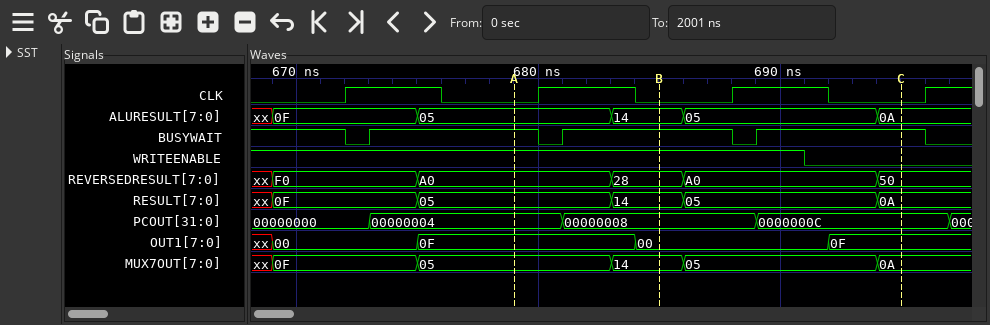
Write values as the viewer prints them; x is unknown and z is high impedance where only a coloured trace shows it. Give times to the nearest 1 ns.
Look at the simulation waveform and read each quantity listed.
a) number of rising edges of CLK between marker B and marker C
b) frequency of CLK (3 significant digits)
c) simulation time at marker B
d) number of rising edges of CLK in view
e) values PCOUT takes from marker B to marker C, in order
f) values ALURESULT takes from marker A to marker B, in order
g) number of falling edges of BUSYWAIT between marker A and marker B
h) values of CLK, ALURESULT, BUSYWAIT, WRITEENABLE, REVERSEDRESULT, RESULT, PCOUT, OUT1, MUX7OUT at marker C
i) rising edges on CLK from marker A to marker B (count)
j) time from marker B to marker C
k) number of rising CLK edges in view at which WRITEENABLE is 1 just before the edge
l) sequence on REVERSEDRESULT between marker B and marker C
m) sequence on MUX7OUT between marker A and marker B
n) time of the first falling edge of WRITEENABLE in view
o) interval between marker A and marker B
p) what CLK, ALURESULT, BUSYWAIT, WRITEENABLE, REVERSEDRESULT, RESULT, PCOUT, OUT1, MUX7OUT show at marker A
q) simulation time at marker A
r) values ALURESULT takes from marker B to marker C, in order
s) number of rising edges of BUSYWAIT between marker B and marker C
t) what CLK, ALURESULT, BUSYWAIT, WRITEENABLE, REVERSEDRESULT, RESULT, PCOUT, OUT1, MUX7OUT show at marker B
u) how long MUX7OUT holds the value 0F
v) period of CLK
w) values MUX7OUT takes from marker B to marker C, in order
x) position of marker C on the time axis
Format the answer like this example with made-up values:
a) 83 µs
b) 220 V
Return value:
a) 1
b) 125 MHz
c) 685 ns
d) 4
e) 00000008, 0000000C
f) 05, 14
g) 1
h) CLK=0, ALURESULT=0A, BUSYWAIT=1, WRITEENABLE=0, REVERSEDRESULT=50, RESULT=0A, PCOUT=0000000C, OUT1=0F, MUX7OUT=0A
i) 1
j) 10 ns
k) 3
l) 28, A0, 50
m) 05, 14
n) 691 ns
o) 6 ns
p) CLK=0, ALURESULT=05, BUSYWAIT=1, WRITEENABLE=1, REVERSEDRESULT=A0, RESULT=05, PCOUT=00000004, OUT1=0F, MUX7OUT=05
q) 679 ns
r) 14, 05, 0A
s) 1
t) CLK=0, ALURESULT=14, BUSYWAIT=1, WRITEENABLE=1, REVERSEDRESULT=28, RESULT=14, PCOUT=00000008, OUT1=00, MUX7OUT=14
u) 6 ns
v) 8 ns
w) 14, 05, 0A
x) 695 ns
